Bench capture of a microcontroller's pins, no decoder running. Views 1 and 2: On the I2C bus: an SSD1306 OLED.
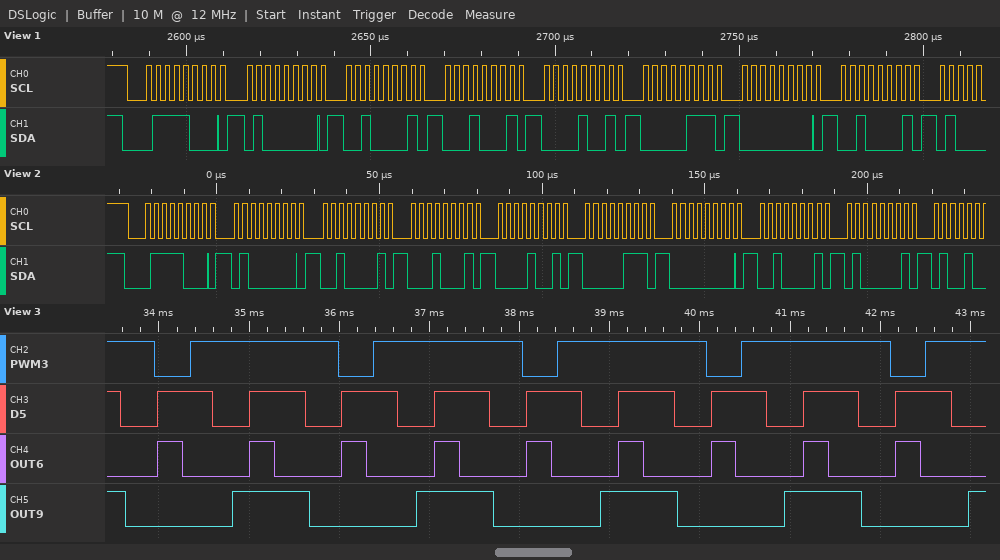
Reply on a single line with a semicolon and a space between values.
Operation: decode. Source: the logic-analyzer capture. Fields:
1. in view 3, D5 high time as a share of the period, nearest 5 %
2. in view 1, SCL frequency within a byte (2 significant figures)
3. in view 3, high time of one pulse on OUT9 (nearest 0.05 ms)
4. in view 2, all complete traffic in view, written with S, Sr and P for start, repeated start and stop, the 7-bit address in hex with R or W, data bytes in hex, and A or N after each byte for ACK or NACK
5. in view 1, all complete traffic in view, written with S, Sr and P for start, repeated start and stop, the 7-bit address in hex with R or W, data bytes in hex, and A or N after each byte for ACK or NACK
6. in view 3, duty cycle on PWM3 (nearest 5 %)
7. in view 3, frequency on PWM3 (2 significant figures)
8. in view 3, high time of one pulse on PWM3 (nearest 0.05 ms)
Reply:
60 %; 400 kHz; 0.85 ms; S 3CW A 40 A 21 A 11 A 09 A 07 A 00 A 21 A 41 A; S 3CW A 40 A 21 A 11 A 09 A 07 A 00 A 21 A; 80 %; 490 Hz; 1.65 ms
